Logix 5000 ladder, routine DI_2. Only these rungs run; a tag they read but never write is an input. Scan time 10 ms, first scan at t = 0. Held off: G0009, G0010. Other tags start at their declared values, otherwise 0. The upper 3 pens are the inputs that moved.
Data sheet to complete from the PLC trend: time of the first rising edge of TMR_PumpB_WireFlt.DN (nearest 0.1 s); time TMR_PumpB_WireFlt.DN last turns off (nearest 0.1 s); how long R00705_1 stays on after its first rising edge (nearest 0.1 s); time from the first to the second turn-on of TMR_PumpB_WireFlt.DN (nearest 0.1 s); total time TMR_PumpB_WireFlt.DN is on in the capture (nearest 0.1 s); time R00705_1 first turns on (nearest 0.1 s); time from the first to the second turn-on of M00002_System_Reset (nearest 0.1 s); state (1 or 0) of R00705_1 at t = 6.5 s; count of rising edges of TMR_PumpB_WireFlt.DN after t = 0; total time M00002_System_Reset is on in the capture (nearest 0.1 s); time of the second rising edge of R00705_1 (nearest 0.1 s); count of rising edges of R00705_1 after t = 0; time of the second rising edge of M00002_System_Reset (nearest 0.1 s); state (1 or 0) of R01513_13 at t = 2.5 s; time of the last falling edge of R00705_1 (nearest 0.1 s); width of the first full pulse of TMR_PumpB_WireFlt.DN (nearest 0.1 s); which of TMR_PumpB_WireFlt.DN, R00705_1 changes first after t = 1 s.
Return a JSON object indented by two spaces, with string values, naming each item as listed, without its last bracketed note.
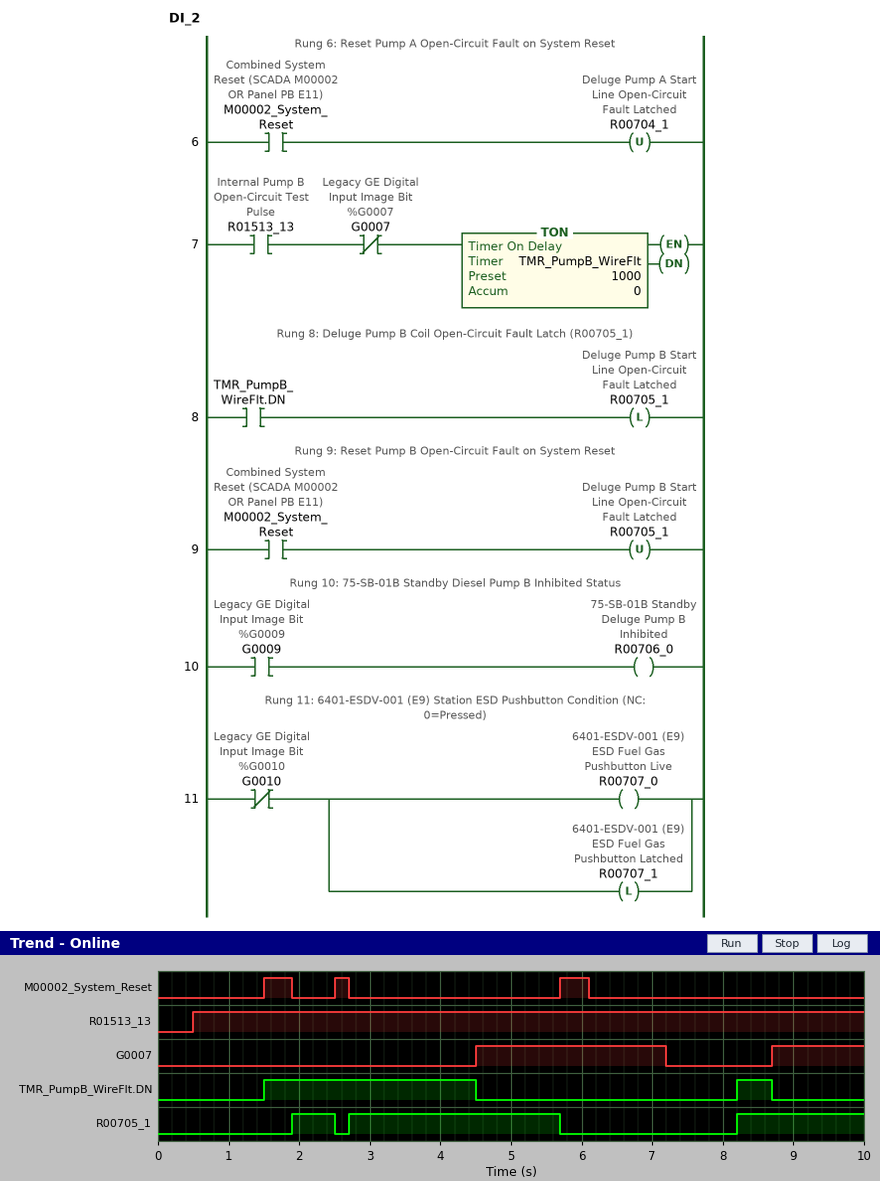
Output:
{
  "time of the first rising edge of TMR_PumpB_WireFlt.DN": "1.5 s",
  "time TMR_PumpB_WireFlt.DN last turns off": "8.7 s",
  "how long R00705_1 stays on after its first rising edge": "0.6 s",
  "time from the first to the second turn-on of TMR_PumpB_WireFlt.DN": "6.7 s",
  "total time TMR_PumpB_WireFlt.DN is on in the capture": "3.5 s",
  "time R00705_1 first turns on": "1.9 s",
  "time from the first to the second turn-on of M00002_System_Reset": "1.0 s",
  "state (1 or 0) of R00705_1 at t = 6.5 s": "0",
  "count of rising edges of TMR_PumpB_WireFlt.DN after t = 0": "2",
  "total time M00002_System_Reset is on in the capture": "1.0 s",
  "time of the second rising edge of R00705_1": "2.7 s",
  "count of rising edges of R00705_1 after t = 0": "3",
  "time of the second rising edge of M00002_System_Reset": "2.5 s",
  "state (1 or 0) of R01513_13 at t = 2.5 s": "1",
  "time of the last falling edge of R00705_1": "5.7 s",
  "width of the first full pulse of TMR_PumpB_WireFlt.DN": "3.0 s",
  "which of TMR_PumpB_WireFlt.DN, R00705_1 changes first after t = 1 s": "TMR_PumpB_WireFlt.DN"
}
